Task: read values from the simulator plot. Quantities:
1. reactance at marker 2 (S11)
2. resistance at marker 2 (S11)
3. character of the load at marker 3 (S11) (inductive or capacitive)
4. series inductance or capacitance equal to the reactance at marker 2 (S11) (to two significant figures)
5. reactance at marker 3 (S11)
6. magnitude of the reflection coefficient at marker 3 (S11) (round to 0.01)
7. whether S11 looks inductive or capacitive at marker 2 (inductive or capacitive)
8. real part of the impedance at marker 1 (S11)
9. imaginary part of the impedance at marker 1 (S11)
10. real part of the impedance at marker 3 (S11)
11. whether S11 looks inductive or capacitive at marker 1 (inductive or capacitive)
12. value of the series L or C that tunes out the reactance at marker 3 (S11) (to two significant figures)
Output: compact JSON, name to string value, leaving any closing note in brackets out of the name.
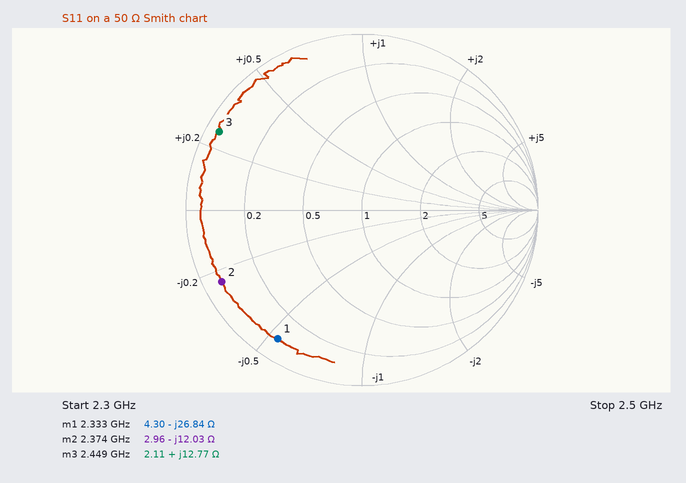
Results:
{"reactance at marker 2": "-12.03 Ω", "resistance at marker 2": "2.96 Ω", "character of the load at marker 3 (S11)": "inductive", "series inductance or capacitance equal to the reactance at marker 2 (S11)": "5.6 pF", "reactance at marker 3": "+12.77 Ω", "magnitude of the reflection coefficient at marker 3 (S11)": "0.92", "whether S11 looks inductive or capacitive at marker 2": "capacitive", "real part of the impedance at marker 1": "4.30 Ω", "imaginary part of the impedance at marker 1": "-26.84 Ω", "real part of the impedance at marker 3": "2.11 Ω", "whether S11 looks inductive or capacitive at marker 1": "capacitive", "value of the series L or C that tunes out the reactance at marker 3 (S11)": "5.1 pF"}
